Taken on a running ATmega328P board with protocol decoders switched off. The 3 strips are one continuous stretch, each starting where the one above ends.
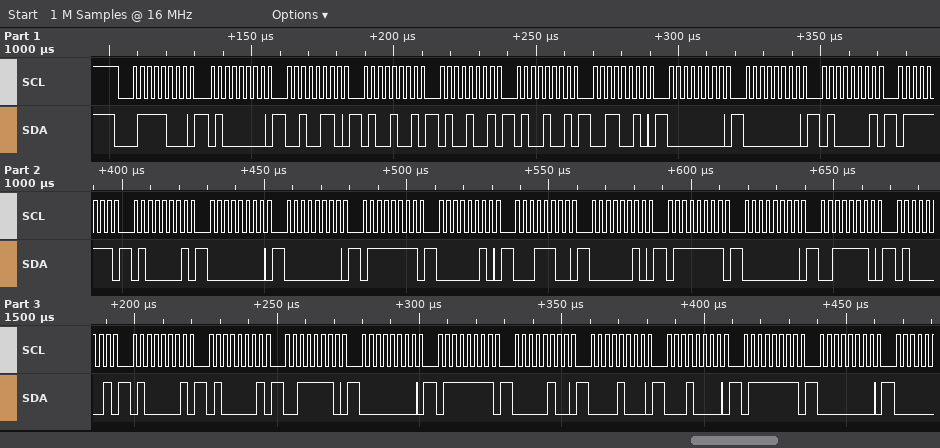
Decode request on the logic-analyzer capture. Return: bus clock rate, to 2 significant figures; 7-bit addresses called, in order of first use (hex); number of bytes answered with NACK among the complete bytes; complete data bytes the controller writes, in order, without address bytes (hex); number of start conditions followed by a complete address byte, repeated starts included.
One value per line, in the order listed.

400 kHz
0x3C
0
40 26 49 49 49 32 00 00 41 7F 41 00 00 7F 02 1C 02 7F 00 3E 41 41 41 3E 00 7F 04 08 10 7F 00
1
